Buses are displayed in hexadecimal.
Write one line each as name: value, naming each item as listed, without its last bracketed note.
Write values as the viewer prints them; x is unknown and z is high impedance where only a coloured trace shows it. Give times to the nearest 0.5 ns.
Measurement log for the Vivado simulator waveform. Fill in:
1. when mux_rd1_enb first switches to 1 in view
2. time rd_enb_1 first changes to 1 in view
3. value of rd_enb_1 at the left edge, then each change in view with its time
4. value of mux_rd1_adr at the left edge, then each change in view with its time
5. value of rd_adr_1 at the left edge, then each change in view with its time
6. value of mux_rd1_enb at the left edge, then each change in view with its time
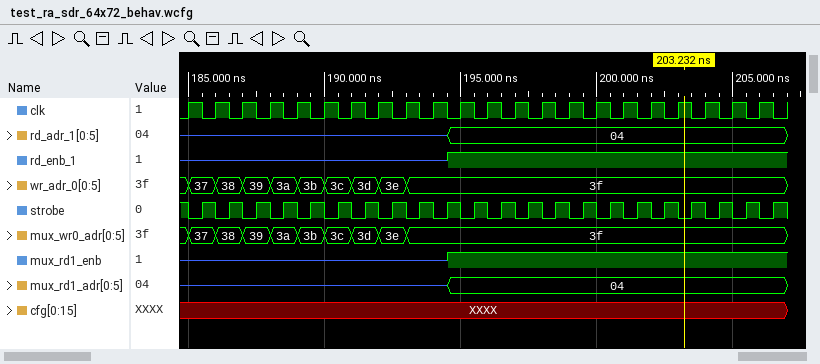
when mux_rd1_enb first switches to 1 in view: 194.5 ns
time rd_enb_1 first changes to 1 in view: 194.5 ns
value of rd_enb_1 at the left edge, then each change in view with its time: z, 1 at 194.5 ns
value of mux_rd1_adr at the left edge, then each change in view with its time: z, 04 at 194.5 ns
value of rd_adr_1 at the left edge, then each change in view with its time: z, 04 at 194.5 ns
value of mux_rd1_enb at the left edge, then each change in view with its time: z, 1 at 194.5 ns
